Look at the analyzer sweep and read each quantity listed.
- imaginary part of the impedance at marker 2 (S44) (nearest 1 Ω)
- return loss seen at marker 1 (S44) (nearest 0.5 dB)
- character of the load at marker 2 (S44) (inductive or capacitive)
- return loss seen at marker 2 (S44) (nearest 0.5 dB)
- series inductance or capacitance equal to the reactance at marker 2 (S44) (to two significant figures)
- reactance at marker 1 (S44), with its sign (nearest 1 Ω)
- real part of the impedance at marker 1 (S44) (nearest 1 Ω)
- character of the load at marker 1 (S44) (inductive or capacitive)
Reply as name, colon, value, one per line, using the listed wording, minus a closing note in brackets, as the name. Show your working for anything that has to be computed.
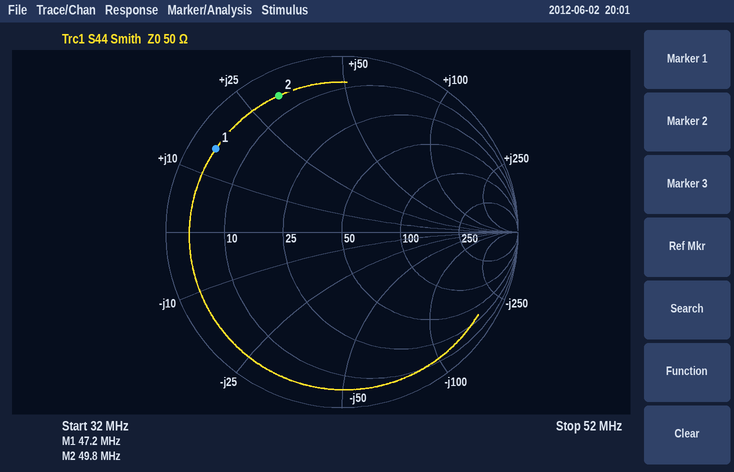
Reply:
imaginary part of the impedance at marker 2 (S44): +32 Ω
return loss seen at marker 1 (S44): 1.5 dB
character of the load at marker 2 (S44): inductive
return loss seen at marker 2 (S44): 1.5 dB
series inductance or capacitance equal to the reactance at marker 2 (S44): L = 32 Ω/(2π × 49.8 MHz) ≈ 102 nH, so 100 nH to two significant figures
reactance at marker 1 (S44), with its sign: +15 Ω
real part of the impedance at marker 1 (S44): 4 Ω
character of the load at marker 1 (S44): inductive
